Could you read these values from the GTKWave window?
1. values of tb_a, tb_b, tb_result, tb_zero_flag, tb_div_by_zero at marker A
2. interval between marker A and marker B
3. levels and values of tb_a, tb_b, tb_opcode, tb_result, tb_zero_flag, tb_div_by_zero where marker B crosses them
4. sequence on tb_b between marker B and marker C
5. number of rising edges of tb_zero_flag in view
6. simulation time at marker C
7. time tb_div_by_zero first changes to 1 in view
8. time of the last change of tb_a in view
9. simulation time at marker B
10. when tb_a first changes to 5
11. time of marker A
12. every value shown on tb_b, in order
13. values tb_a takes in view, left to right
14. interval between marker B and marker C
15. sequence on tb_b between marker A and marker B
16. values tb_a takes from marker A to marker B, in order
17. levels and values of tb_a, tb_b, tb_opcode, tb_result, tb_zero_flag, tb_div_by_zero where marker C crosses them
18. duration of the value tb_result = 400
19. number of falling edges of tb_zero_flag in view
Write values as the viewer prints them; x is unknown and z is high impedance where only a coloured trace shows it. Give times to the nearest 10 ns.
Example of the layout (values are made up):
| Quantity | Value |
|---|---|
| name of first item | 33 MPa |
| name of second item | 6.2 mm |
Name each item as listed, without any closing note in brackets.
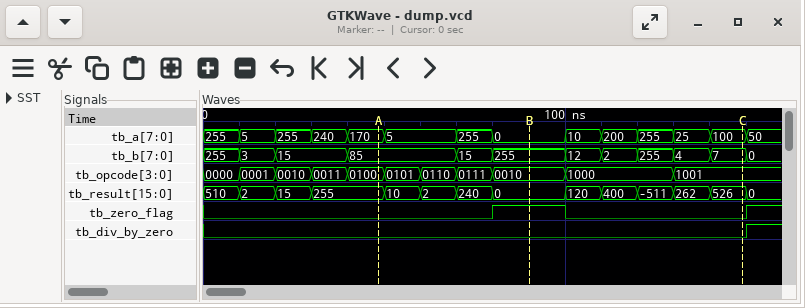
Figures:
| Quantity | Value |
|---|---|
| values of tb_a, tb_b, tb_result, tb_zero_flag, tb_div_by_zero at marker A | tb_a=170, tb_b=85, tb_result=255, tb_zero_flag=0, tb_div_by_zero=0 |
| interval between marker A and marker B | 40 ns |
| levels and values of tb_a, tb_b, tb_opcode, tb_result, tb_zero_flag, tb_div_by_zero where marker B crosses them | tb_a=0, tb_b=255, tb_opcode=0010, tb_result=0, tb_zero_flag=1, tb_div_by_zero=0 |
| sequence on tb_b between marker B and marker C | 255, 12, 2, 255, 4, 7 |
| number of rising edges of tb_zero_flag in view | 2 |
| simulation time at marker C | 150 ns |
| time tb_div_by_zero first changes to 1 in view | 150 ns |
| time of the last change of tb_a in view | 150 ns |
| simulation time at marker B | 90 ns |
| when tb_a first changes to 5 | 10 ns |
| time of marker A | 50 ns |
| every value shown on tb_b, in order | 255, 3, 15, 85, 15, 255, 12, 2, 255, 4, 7, 0 |
| values tb_a takes in view, left to right | 255, 5, 255, 240, 170, 5, 255, 0, 10, 200, 255, 25, 100, 50 |
| interval between marker B and marker C | 60 ns |
| sequence on tb_b between marker A and marker B | 85, 15, 255 |
| values tb_a takes from marker A to marker B, in order | 170, 5, 255, 0 |
| levels and values of tb_a, tb_b, tb_opcode, tb_result, tb_zero_flag, tb_div_by_zero where marker C crosses them | tb_a=100, tb_b=7, tb_opcode=1001, tb_result=526, tb_zero_flag=0, tb_div_by_zero=0 |
| duration of the value tb_result = 400 | 10 ns |
| number of falling edges of tb_zero_flag in view | 1 |
